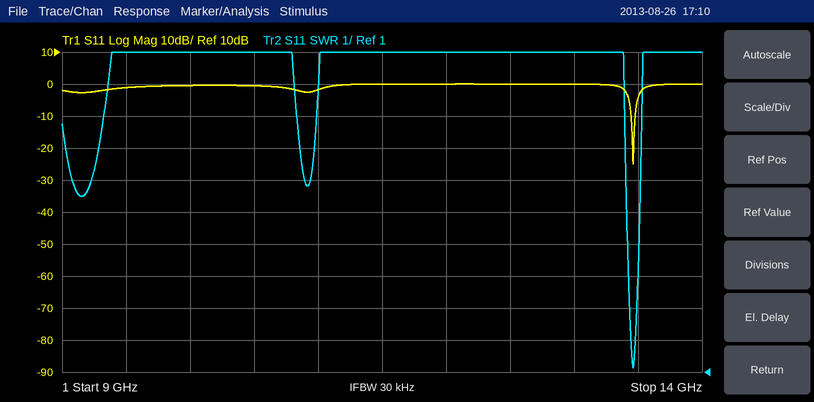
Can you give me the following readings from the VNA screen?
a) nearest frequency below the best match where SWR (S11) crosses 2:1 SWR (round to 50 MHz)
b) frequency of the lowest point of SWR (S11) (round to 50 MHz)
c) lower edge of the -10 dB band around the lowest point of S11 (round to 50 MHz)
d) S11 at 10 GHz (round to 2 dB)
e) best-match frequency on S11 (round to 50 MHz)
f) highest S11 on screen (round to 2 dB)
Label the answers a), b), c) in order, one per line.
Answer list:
a) 13.45 GHz
b) 13.45 GHz
c) 13.45 GHz
d) 0 dB
e) 13.45 GHz
f) 0 dB
